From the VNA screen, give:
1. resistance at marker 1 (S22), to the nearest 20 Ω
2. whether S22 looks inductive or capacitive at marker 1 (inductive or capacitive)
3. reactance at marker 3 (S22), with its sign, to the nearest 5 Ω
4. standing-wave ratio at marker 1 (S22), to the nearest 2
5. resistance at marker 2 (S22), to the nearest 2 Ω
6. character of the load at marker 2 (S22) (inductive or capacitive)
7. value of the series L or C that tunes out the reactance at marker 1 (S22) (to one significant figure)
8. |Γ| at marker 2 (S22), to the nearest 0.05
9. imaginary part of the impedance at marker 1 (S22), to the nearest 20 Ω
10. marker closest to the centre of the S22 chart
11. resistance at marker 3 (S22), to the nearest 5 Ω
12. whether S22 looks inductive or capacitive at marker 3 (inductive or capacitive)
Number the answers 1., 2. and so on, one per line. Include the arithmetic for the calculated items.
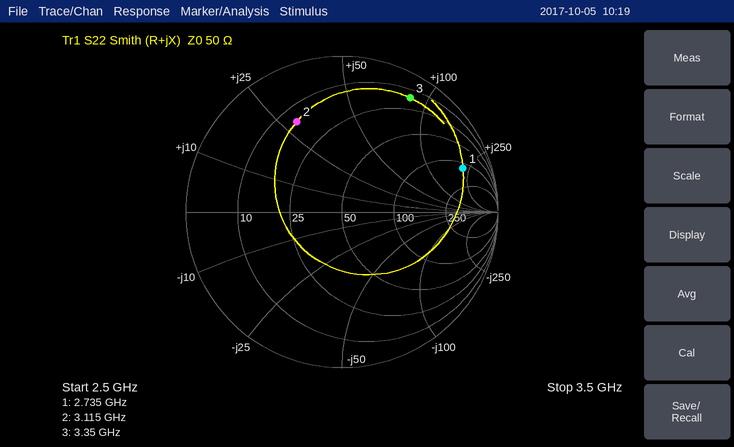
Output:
1. 120 Ω
2. inductive
3. +85 Ω
4. 10
5. 14 Ω
6. inductive
7. C = 1/(2π × 2.735 GHz × 220 Ω) ≈ 265 fF, so 300 fF to one significant figure
8. 0.65
9. +220 Ω
10. marker 2
11. 15 Ω
12. inductive
